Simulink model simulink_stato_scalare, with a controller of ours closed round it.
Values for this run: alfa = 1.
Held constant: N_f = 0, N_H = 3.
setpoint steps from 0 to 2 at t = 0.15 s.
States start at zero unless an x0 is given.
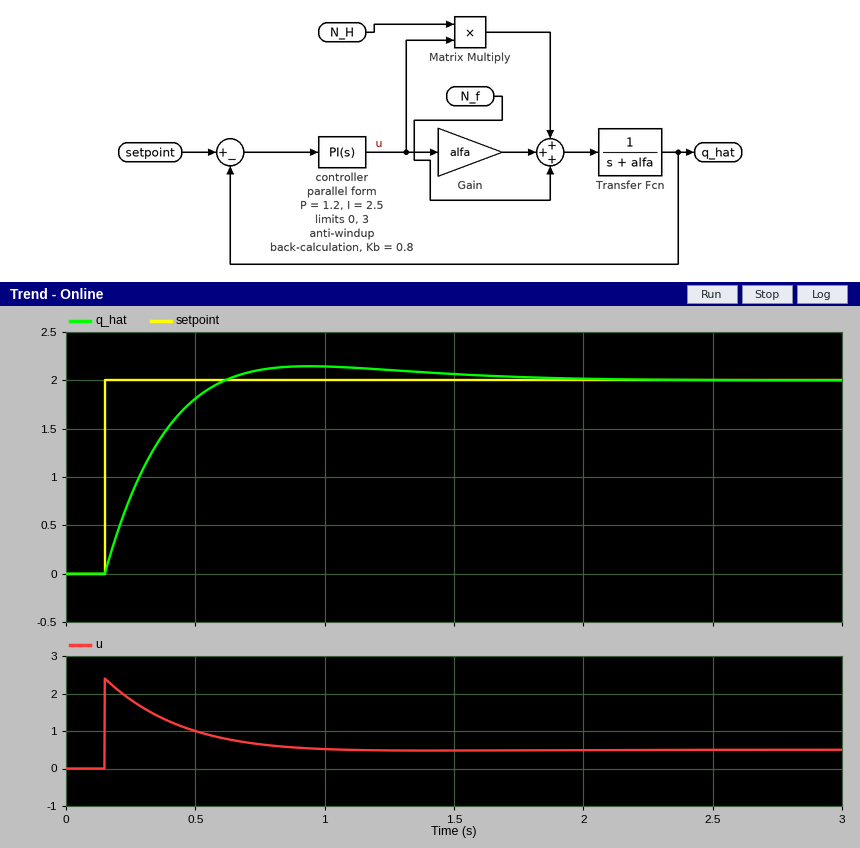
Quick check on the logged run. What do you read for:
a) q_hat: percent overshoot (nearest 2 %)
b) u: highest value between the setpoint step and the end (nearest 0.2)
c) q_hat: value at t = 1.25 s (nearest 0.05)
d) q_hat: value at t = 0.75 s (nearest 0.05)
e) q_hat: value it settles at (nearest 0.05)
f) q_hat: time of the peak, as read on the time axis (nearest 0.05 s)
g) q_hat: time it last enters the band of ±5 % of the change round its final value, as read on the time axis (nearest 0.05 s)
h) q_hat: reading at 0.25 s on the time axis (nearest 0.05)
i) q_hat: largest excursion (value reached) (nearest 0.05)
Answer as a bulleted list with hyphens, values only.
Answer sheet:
- 8 %
- 2.4
- 2.10
- 2.10
- 2.00
- 0.95 s
- 1.30 s
- 0.80
- 2.15
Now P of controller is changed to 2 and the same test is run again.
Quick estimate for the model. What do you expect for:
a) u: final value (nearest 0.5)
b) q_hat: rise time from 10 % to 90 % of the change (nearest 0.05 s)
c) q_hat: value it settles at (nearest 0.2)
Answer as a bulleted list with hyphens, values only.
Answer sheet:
- 0.5
- 0.25 s
- 2.0
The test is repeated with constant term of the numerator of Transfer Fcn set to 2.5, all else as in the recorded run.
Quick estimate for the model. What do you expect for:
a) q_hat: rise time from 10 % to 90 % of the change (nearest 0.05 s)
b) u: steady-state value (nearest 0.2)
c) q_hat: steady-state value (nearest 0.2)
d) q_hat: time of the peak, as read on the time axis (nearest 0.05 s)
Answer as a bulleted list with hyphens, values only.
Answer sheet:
- 0.15 s
- 0.2
- 2.0
- 0.55 s
